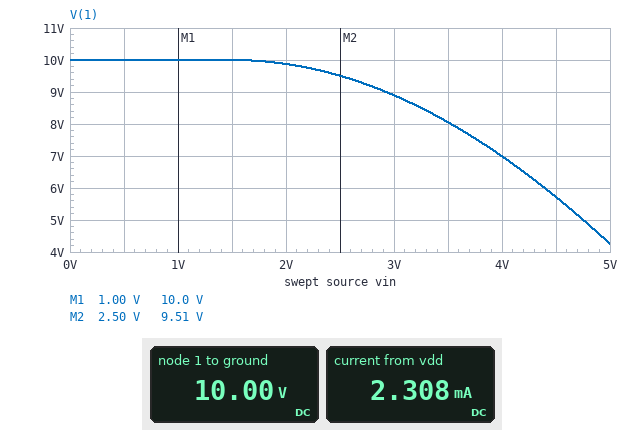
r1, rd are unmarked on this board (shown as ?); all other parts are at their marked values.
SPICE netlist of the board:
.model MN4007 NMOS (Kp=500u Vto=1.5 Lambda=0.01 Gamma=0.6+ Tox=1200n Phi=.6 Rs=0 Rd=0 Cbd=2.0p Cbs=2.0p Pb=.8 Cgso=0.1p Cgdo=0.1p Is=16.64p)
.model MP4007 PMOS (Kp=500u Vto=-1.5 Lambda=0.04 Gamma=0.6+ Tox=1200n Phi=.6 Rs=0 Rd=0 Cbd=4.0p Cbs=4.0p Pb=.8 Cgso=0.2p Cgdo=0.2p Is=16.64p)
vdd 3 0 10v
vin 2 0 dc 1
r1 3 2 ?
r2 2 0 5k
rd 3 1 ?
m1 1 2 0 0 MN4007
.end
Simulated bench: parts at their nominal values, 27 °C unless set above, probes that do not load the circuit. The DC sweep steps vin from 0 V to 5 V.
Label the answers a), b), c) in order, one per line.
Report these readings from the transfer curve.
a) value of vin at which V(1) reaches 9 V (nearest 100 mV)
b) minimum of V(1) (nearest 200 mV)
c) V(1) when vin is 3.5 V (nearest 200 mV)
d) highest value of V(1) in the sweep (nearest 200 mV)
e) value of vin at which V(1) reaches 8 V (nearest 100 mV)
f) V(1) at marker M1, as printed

a) 2.9 V
b) 4.2 V
c) 8.0 V
d) 10.0 V
e) 3.5 V
f) 10.0 V
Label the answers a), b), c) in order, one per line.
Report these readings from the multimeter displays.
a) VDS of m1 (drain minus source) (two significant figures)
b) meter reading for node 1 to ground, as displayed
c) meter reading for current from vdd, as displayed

a) 10 V
b) 10.00 V
c) 2.308 mA
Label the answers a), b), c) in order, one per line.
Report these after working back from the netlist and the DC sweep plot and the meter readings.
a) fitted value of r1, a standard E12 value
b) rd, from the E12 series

a) 3.9 kΩ
b) 1.8 kΩ
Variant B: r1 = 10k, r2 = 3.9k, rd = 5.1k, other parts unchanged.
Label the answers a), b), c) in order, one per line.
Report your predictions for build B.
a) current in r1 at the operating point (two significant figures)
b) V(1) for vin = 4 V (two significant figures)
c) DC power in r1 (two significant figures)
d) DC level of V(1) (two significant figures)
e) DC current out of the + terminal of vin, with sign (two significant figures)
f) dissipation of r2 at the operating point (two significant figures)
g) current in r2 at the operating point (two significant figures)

a) 900 µA
b) 2.1 V
c) 8.1 mW
d) 10 V
e) -640 µA
f) 260 µW
g) 260 µA
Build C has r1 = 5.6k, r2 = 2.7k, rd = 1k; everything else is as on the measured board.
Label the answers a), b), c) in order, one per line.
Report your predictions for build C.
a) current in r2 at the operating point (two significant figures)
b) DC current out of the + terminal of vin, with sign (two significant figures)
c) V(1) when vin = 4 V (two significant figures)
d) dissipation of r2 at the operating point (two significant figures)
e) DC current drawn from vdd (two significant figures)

a) 370 µA
b) -1.2 mA
c) 8.3 V
d) 370 µW
e) 1.6 mA
